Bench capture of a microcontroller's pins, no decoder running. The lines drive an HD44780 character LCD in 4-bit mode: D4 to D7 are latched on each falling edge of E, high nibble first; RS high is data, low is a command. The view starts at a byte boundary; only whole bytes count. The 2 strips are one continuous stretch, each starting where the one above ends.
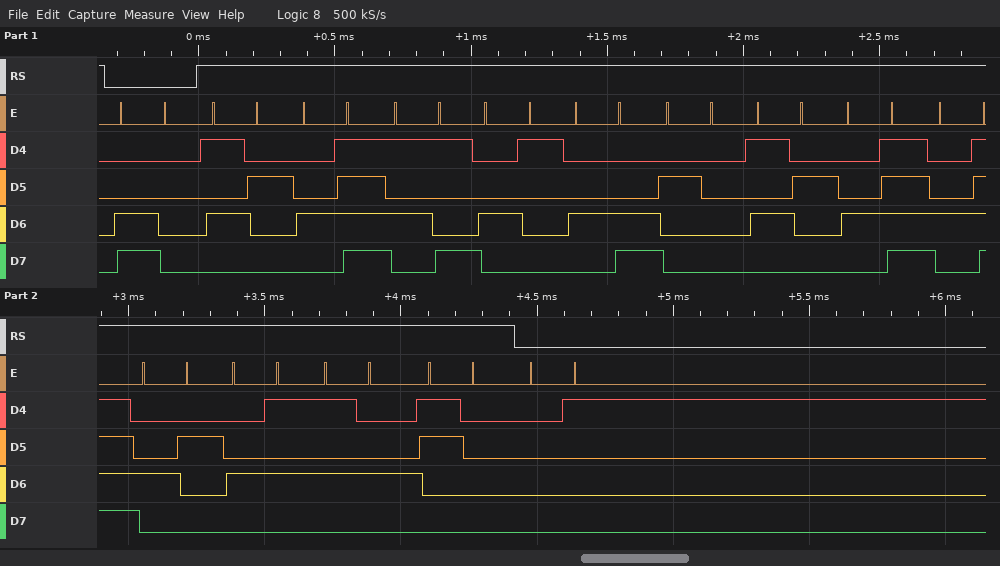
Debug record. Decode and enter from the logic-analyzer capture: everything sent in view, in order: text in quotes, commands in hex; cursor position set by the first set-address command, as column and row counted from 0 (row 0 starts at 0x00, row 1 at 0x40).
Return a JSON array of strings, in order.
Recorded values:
["0xC0 \"ROYAL ROOBET0\" 0x01", "column 0, row 1"]
